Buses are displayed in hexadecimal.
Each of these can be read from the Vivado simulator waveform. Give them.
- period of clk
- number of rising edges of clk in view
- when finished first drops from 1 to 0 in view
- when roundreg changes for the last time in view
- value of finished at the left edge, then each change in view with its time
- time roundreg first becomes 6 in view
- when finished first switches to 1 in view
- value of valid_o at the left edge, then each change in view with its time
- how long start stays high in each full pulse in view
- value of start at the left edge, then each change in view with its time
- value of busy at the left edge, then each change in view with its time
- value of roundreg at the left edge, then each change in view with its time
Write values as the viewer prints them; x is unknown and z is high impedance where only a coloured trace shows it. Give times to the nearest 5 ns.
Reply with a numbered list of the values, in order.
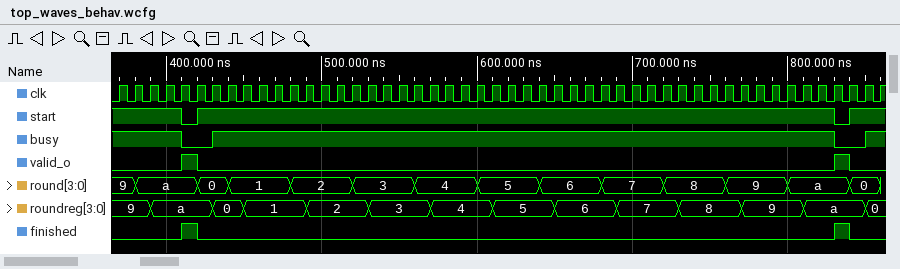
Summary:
1. 10 ns
2. 50
3. 420 ns
4. 850 ns
5. 0, 1 at 410 ns, 0 at 420 ns, 1 at 830 ns, 0 at 840 ns
6. 650 ns
7. 410 ns
8. 0, 1 at 410 ns, 0 at 420 ns, 1 at 830 ns, 0 at 840 ns
9. 410 ns
10. 1, 0 at 410 ns, 1 at 420 ns, 0 at 830 ns, 1 at 840 ns
11. 1, 0 at 410 ns, 1 at 430 ns, 0 at 830 ns, 1 at 850 ns
12. 9, a at 390 ns, 0 at 430 ns, 1 at 450 ns, 2 at 490 ns, 3 at 530 ns, 4 at 570 ns, 5 at 610 ns, 6 at 650 ns, 7 at 690 ns, 8 at 730 ns, 9 at 770 ns, a at 810 ns, 0 at 850 ns
